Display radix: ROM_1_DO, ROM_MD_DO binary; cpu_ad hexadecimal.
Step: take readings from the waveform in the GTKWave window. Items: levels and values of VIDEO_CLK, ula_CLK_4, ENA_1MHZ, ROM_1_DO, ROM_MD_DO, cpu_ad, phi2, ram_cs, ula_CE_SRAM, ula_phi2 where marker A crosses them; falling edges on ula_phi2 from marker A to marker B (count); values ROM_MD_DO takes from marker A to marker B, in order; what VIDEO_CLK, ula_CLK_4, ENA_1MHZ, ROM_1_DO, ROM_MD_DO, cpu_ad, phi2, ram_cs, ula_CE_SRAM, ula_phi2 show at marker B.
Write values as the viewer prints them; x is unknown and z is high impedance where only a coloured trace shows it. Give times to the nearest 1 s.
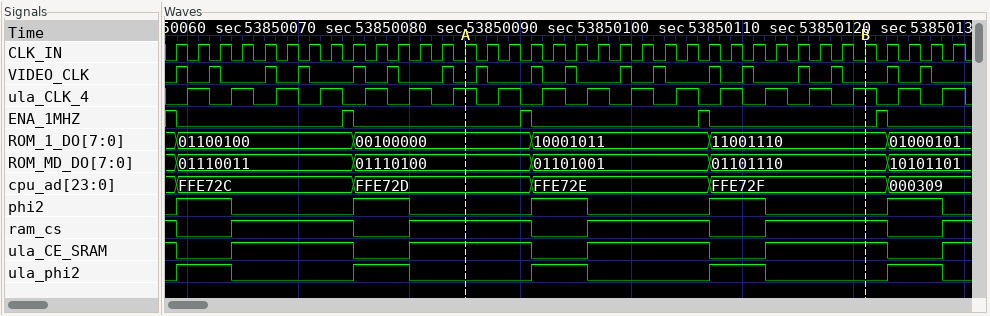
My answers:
VIDEO_CLK=0, ula_CLK_4=1, ENA_1MHZ=0, ROM_1_DO=00100000, ROM_MD_DO=01110100, cpu_ad=FFE72D, phi2=0, ram_cs=1, ula_CE_SRAM=1, ula_phi2=0
2
01110100, 01101001, 01101110
VIDEO_CLK=0, ula_CLK_4=1, ENA_1MHZ=0, ROM_1_DO=11001110, ROM_MD_DO=01101110, cpu_ad=FFE72F, phi2=0, ram_cs=1, ula_CE_SRAM=1, ula_phi2=0
